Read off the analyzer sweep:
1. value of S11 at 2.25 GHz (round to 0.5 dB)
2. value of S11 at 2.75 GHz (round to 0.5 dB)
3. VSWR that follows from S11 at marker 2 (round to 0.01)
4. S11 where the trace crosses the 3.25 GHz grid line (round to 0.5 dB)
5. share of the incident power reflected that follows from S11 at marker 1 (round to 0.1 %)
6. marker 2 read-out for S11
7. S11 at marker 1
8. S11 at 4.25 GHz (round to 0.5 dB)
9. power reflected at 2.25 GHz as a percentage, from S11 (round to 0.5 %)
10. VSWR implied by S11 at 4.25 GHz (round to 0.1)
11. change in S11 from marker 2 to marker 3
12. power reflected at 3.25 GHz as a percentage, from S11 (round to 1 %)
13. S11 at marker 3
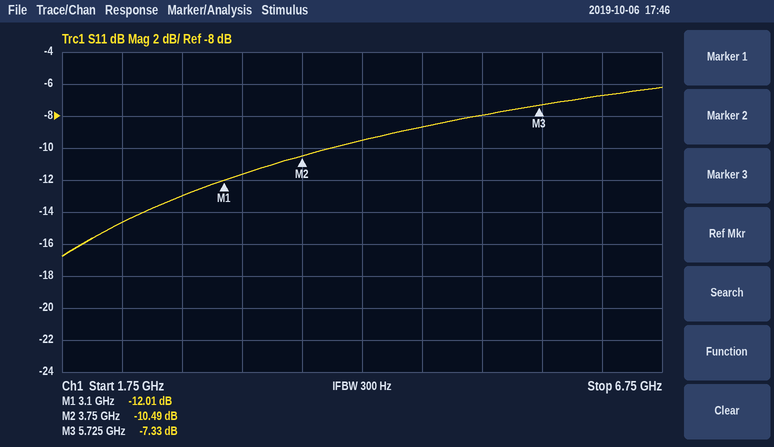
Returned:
-14.5 dB
-13.0 dB
1.85
-11.5 dB
6.3 %
-10.49 dB
-12.01 dB
-9.5 dB
3.5 %
2.0
3.16 dB
7 %
-7.33 dB
